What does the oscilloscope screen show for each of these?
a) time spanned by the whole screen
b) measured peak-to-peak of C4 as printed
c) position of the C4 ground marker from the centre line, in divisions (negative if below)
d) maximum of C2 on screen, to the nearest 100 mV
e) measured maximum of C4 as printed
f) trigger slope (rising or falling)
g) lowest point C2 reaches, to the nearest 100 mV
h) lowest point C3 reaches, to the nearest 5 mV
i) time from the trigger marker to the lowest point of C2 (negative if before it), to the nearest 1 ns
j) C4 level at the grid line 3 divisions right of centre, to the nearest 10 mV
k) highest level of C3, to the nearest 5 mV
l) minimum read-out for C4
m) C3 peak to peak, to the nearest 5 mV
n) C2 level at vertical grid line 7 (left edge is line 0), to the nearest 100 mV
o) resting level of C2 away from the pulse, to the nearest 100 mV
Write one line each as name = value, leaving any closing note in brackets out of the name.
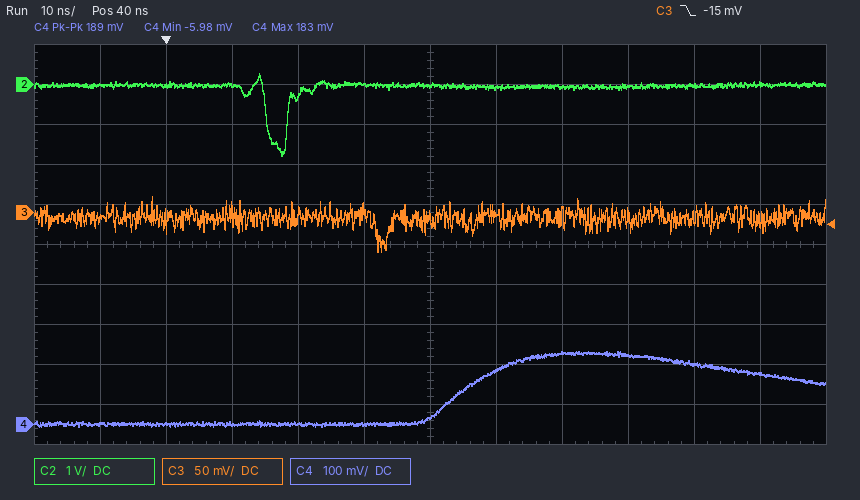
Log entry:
time spanned by the whole screen = 120 ns
measured peak-to-peak of C4 as printed = 189 mV
position of the C4 ground marker from the centre line, in divisions = -4.5 div
maximum of C2 on screen, to the nearest 100 mV = 300 mV
measured maximum of C4 as printed = 183 mV
trigger slope = falling
lowest point C2 reaches, to the nearest 100 mV = -1.8 V
lowest point C3 reaches, to the nearest 5 mV = -50 mV
time from the trigger marker to the lowest point of C2 (negative if before it), to the nearest 1 ns = +18 ns
C4 level at the grid line 3 divisions right of centre, to the nearest 10 mV = 170 mV
highest level of C3, to the nearest 5 mV = 20 mV
minimum read-out for C4 = -5.98 mV
C3 peak to peak, to the nearest 5 mV = 70 mV
C2 level at vertical grid line 7 (left edge is line 0), to the nearest 100 mV = -100 mV
resting level of C2 away from the pulse, to the nearest 100 mV = 0.0 V
